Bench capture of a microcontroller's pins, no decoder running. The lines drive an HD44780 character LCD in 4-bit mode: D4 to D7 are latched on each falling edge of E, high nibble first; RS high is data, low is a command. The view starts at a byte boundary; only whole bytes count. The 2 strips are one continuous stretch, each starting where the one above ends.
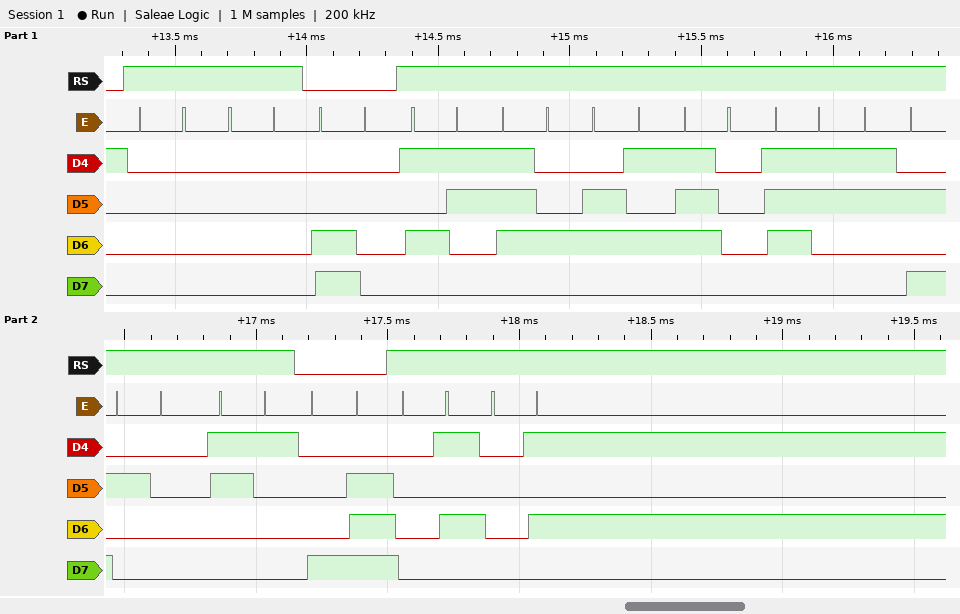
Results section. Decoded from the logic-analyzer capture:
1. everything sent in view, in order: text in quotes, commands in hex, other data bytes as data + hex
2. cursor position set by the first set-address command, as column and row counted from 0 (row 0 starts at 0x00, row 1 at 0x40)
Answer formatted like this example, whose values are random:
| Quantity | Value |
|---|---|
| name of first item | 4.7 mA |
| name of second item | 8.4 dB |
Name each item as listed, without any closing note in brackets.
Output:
| Quantity | Value |
|---|---|
| everything sent in view, in order: text in quotes, commands in hex, other data bytes as data + hex | data 00 00 0xC0 "Steps: 1" 0x8E data 05 05 |
| cursor position set by the first set-address command, as column and row counted from 0 | column 0, row 1 |
